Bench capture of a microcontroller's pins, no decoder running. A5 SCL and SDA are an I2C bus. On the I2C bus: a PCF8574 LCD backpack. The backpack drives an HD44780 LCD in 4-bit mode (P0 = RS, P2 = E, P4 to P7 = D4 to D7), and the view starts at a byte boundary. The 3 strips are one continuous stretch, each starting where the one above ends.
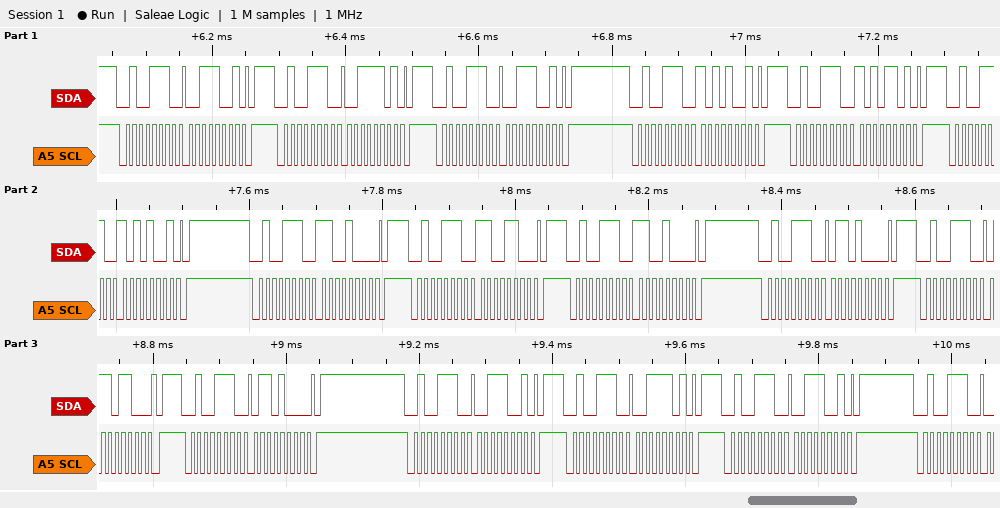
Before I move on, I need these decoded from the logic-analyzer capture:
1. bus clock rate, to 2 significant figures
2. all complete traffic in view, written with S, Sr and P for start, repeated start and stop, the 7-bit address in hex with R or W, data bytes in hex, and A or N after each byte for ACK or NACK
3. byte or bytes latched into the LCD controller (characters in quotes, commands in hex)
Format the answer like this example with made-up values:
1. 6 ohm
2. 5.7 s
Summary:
1. 100 kHz
2. S 27W A 39 A P S 27W A 3D A P S 27W A 39 A P S 27W A A9 A P S 27W A AD A P S 27W A A9 A P S 27W A C8 A P S 27W A CC A P S 27W A C8 A P S 27W A 68 A P S 27W A 6C A P S 27W A 68 A P S 27W A 39 A P S 27W A 3D A P S 27W A 39 A P S 27W A
3. ':' 0xC6
